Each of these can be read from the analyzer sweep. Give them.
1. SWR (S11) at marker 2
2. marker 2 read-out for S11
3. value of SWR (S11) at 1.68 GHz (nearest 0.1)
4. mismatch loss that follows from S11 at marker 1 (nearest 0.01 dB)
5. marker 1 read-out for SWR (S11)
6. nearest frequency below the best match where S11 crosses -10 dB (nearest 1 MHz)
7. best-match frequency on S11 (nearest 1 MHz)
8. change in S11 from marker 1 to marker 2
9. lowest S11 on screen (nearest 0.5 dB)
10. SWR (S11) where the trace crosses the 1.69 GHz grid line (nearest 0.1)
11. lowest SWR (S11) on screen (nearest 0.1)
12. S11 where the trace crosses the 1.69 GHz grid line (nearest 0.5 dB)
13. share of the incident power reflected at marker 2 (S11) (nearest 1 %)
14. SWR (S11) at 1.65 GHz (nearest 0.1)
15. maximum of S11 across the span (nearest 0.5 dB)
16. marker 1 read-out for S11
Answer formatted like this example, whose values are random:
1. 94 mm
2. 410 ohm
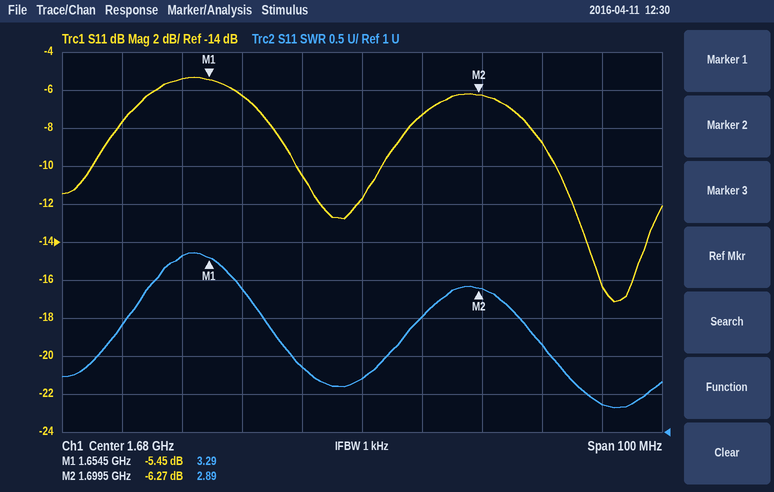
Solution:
1. 2.89
2. -6.27 dB
3. 1.7
4. 1.46 dB
5. 3.29
6. 1.712 GHz
7. 1.722 GHz
8. -0.82 dB
9. -17.0 dB
10. 2.5
11. 1.3
12. -7.5 dB
13. 24 %
14. 3.3
15. -5.5 dB
16. -5.45 dB
